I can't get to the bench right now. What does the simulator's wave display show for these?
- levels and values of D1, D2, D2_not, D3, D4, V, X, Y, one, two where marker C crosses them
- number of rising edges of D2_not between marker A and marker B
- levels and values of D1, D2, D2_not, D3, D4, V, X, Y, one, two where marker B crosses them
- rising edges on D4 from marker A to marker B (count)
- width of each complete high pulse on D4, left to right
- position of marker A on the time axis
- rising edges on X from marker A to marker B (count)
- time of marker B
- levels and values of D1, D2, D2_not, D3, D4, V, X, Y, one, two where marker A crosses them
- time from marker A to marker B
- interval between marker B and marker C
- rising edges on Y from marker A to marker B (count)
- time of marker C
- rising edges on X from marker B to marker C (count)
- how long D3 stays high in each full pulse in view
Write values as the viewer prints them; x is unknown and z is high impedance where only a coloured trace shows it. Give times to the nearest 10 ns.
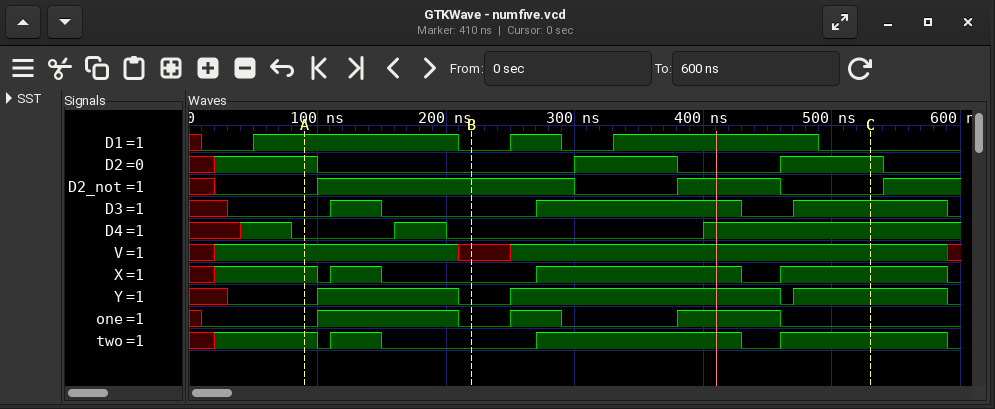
D1=0, D2=1, D2_not=0, D3=1, D4=1, V=1, X=1, Y=1, one=0, two=1
1
D1=0, D2=0, D2_not=1, D3=0, D4=0, V=x, X=0, Y=0, one=0, two=0
1
40 ns
90 ns
1
220 ns
D1=1, D2=1, D2_not=0, D3=0, D4=0, V=1, X=1, Y=0, one=0, two=1
130 ns
310 ns
1
530 ns
2
40 ns, 160 ns, 120 ns
